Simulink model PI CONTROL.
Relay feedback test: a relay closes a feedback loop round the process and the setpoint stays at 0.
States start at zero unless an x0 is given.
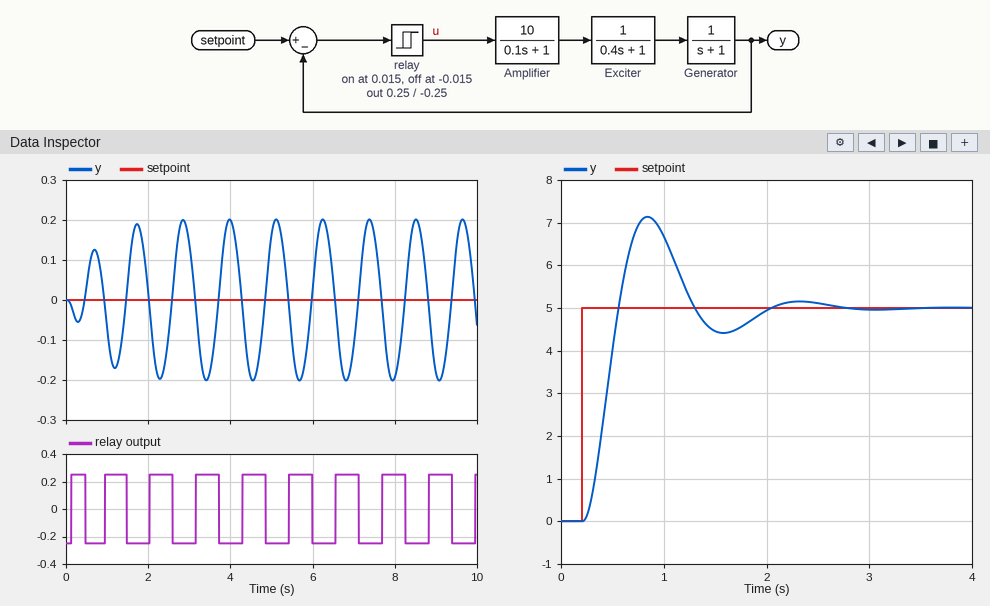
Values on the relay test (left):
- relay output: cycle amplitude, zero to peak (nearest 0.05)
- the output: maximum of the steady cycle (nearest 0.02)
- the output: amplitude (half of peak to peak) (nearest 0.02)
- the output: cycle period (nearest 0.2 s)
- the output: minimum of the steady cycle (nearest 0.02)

0.25
0.20
0.20
1.2 s
-0.20
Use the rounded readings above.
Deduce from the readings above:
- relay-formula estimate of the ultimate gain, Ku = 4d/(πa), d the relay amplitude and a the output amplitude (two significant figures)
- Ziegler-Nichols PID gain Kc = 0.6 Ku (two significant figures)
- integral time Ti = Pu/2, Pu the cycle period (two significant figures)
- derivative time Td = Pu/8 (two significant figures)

1.6
0.96
0.60 s
0.15 s
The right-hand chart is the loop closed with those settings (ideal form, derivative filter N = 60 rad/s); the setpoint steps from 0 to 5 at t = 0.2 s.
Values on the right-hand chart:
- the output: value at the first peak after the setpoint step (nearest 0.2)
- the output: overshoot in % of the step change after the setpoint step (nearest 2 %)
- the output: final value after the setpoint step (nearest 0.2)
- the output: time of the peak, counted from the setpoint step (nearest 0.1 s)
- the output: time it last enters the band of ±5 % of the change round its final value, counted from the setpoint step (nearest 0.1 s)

7.2
42 %
5.0
0.6 s
1.7 s
